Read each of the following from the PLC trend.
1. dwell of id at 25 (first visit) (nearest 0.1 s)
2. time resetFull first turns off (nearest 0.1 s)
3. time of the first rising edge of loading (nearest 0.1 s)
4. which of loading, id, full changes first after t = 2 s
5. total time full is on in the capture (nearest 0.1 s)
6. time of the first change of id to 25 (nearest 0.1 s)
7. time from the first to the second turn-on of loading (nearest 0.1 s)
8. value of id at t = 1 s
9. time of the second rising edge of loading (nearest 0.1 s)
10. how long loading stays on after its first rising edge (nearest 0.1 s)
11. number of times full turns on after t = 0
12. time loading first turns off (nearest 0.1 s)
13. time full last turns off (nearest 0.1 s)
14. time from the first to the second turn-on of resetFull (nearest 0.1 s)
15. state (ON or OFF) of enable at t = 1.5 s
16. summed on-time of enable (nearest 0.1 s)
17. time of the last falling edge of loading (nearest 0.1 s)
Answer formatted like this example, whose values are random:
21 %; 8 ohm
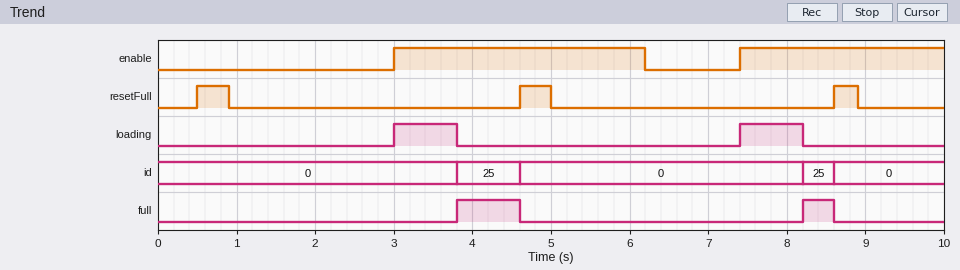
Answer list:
0.8 s; 0.9 s; 3.0 s; loading; 1.2 s; 3.8 s; 4.4 s; 0; 7.4 s; 0.8 s; 2; 3.8 s; 8.6 s; 4.1 s; OFF; 5.8 s; 8.2 s
